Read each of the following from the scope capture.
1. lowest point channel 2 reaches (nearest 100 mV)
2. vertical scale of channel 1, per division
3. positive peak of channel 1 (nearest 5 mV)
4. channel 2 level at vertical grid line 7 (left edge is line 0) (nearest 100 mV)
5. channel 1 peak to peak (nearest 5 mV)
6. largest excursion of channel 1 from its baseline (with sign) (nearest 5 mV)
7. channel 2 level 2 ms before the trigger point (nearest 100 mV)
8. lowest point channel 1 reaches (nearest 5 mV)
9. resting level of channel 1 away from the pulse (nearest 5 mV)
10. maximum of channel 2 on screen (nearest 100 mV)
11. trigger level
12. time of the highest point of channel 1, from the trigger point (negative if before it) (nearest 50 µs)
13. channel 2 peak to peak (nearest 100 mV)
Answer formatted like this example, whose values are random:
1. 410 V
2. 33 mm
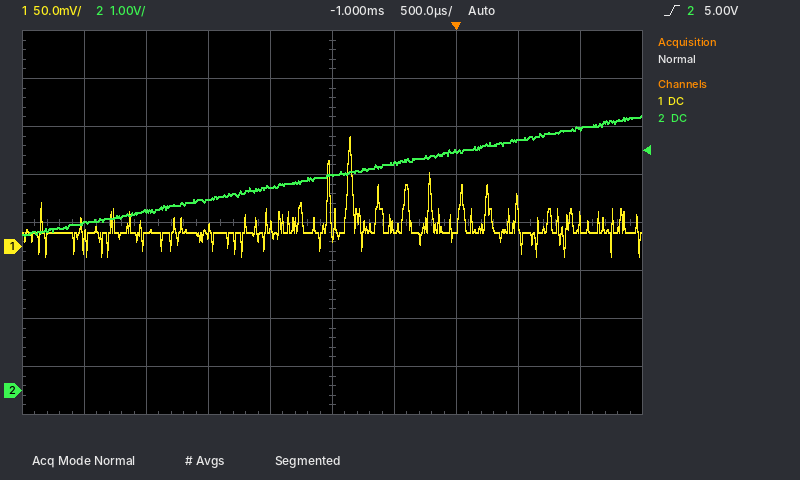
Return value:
1. 3.2 V
2. 50 mV
3. 115 mV
4. 5.0 V
5. 125 mV
6. +100 mV
7. 4.0 V
8. -10 mV
9. 15 mV
10. 5.7 V
11. 5.00 V
12. -850 µs
13. 2.5 V
